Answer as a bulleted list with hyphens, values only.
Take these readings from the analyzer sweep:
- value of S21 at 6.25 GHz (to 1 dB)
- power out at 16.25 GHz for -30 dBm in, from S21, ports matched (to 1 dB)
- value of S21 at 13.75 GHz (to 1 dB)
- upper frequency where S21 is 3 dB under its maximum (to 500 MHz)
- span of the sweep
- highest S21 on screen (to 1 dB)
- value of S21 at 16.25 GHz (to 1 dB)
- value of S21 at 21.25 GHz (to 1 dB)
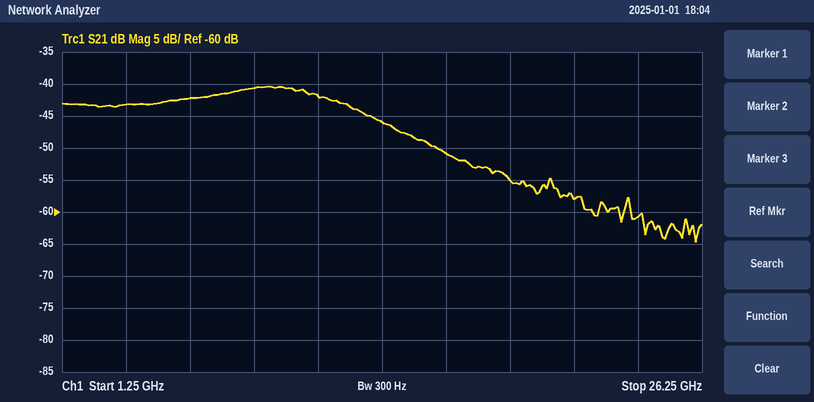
- -42 dB
- -81 dBm
- -46 dB
- 12.5 GHz
- 25 GHz
- -40 dB
- -51 dB
- -58 dB
